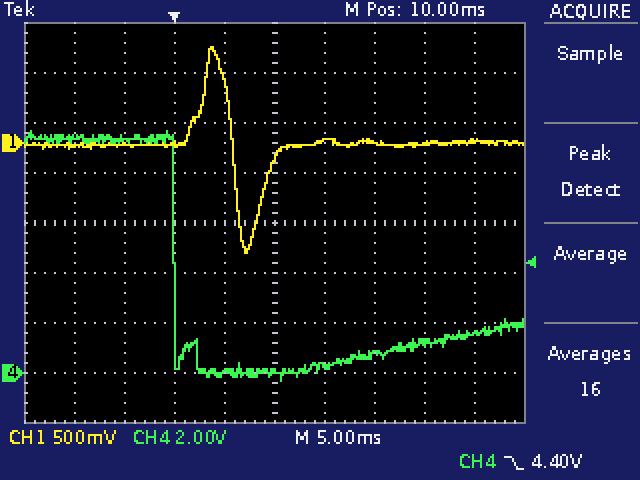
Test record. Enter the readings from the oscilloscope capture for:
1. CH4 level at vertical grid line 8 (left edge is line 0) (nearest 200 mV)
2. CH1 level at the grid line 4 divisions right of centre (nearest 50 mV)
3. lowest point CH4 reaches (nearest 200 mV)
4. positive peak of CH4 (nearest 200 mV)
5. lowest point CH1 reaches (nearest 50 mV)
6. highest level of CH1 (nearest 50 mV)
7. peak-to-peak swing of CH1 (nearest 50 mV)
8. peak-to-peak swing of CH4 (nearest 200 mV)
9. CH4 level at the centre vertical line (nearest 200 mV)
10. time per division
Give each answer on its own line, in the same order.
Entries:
1.2 V
0 mV
-400 mV
9.6 V
-1.10 V
950 mV
2.05 V
10.0 V
0.0 V
5 ms
